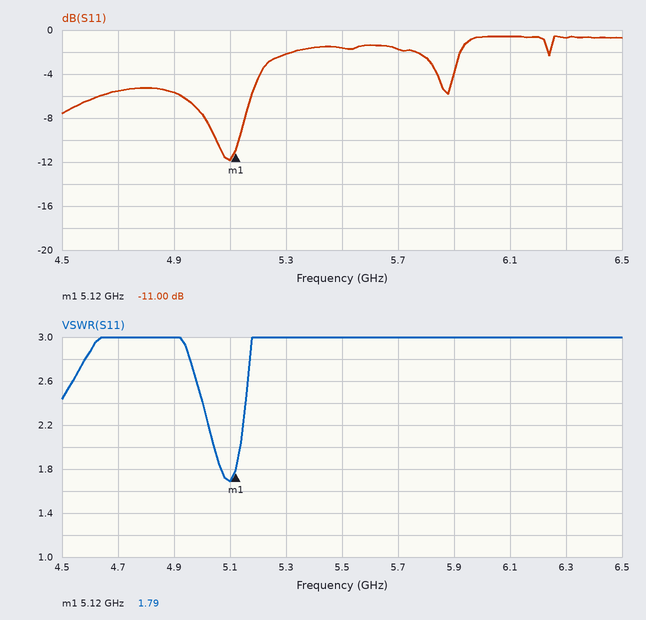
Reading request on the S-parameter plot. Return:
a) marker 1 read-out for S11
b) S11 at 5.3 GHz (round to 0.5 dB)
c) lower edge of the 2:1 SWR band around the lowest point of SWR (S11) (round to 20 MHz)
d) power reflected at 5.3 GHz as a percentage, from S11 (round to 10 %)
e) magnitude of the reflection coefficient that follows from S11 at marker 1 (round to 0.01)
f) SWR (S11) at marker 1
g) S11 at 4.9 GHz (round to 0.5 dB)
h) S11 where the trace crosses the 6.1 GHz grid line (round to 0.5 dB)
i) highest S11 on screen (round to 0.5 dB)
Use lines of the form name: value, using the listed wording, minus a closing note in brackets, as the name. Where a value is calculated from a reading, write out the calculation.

marker 1 read-out for S11: -11.00 dB
S11 at 5.3 GHz: -2.0 dB
lower edge of the 2:1 SWR band around the lowest point of SWR (S11): 5.04 GHz
power reflected at 5.3 GHz as a percentage, from S11: 10^(-2/10) ≈ 63.1 %, so 60 % to the nearest 10 %
magnitude of the reflection coefficient that follows from S11 at marker 1: 10^(-11/20) ≈ 0.28
SWR (S11) at marker 1: 1.79
S11 at 4.9 GHz: -5.5 dB
S11 where the trace crosses the 6.1 GHz grid line: -0.5 dB
highest S11 on screen: -0.5 dB
